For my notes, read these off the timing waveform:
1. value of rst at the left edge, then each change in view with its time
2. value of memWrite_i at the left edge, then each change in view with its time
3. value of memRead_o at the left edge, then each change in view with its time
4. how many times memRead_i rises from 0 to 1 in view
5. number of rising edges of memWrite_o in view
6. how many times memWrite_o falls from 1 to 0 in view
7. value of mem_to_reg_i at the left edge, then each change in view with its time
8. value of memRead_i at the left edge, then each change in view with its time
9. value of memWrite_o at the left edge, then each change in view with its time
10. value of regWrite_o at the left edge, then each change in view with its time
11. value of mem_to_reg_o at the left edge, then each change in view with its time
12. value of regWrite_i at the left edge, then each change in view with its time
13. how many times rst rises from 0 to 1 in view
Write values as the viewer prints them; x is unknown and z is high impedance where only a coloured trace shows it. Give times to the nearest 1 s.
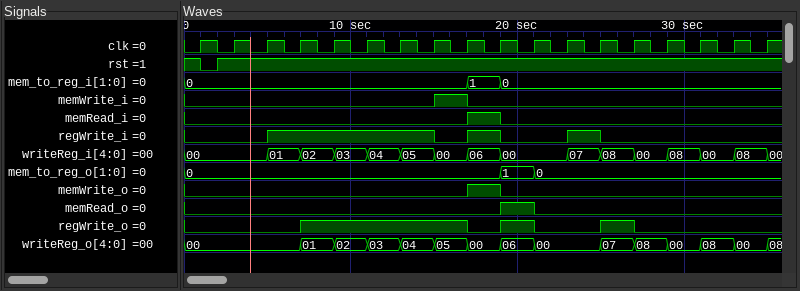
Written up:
1, 0 at 1 s, 1 at 2 s
0, 1 at 15 s, 0 at 17 s
0, 1 at 19 s, 0 at 21 s
1
1
1
0, 1 at 17 s, 0 at 19 s
0, 1 at 17 s, 0 at 19 s
0, 1 at 17 s, 0 at 19 s
0, 1 at 7 s, 0 at 17 s, 1 at 19 s, 0 at 21 s, 1 at 25 s, 0 at 27 s
0, 1 at 19 s, 0 at 21 s
0, 1 at 5 s, 0 at 15 s, 1 at 17 s, 0 at 19 s, 1 at 23 s, 0 at 25 s
1
